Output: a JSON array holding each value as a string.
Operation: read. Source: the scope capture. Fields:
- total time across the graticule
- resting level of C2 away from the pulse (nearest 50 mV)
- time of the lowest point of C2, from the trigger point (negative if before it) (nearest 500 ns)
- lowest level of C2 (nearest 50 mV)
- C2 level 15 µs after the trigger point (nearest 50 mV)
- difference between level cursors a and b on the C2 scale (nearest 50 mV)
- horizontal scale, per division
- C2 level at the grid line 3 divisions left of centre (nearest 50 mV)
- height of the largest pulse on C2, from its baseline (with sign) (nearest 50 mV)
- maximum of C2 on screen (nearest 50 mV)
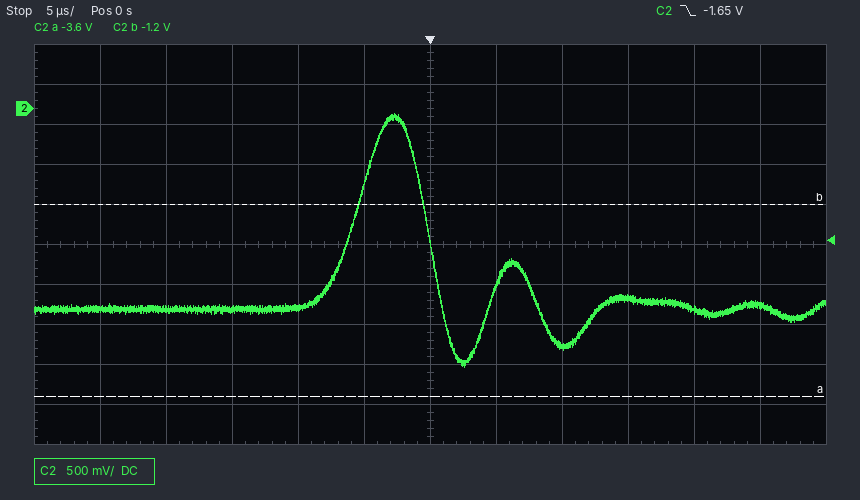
["60 µs", "-2.50 V", "+2.5 µs", "-3.25 V", "-2.35 V", "2.40 V", "5 µs", "-2.50 V", "+2.45 V", "-50 mV"]
